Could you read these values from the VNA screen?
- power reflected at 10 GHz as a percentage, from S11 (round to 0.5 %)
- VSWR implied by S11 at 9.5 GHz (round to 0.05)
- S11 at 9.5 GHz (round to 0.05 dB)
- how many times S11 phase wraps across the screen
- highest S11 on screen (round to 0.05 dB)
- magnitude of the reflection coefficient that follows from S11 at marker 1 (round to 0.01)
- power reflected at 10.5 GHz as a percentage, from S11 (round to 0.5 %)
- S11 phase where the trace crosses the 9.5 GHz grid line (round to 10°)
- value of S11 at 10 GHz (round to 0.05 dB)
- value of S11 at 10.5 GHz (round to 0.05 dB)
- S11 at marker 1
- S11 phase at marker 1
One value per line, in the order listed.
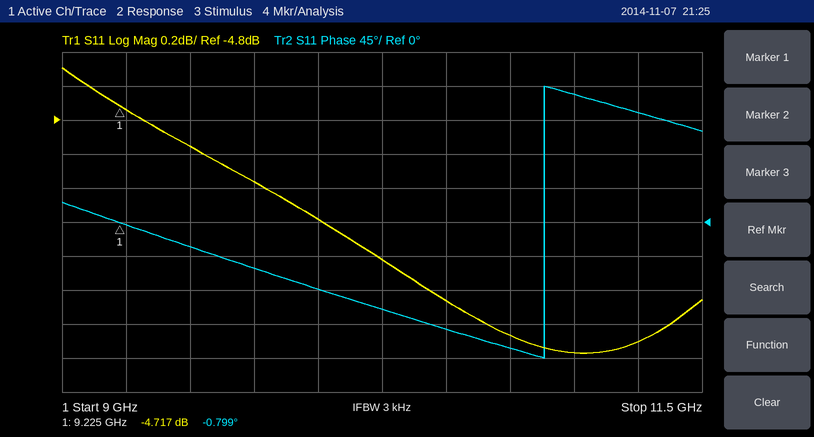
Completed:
29.0 %
3.60
-4.95 dB
1
-4.50 dB
0.58
26.0 %
-30°
-5.40 dB
-5.85 dB
-4.717 dB
-0.799°
